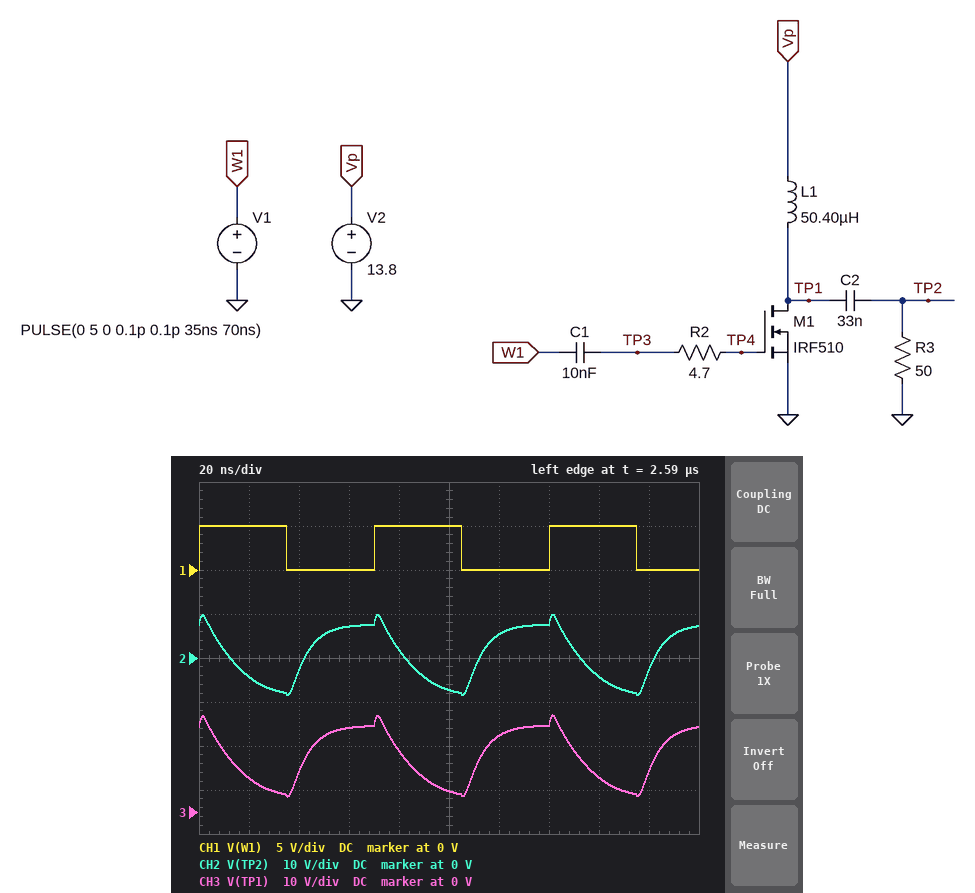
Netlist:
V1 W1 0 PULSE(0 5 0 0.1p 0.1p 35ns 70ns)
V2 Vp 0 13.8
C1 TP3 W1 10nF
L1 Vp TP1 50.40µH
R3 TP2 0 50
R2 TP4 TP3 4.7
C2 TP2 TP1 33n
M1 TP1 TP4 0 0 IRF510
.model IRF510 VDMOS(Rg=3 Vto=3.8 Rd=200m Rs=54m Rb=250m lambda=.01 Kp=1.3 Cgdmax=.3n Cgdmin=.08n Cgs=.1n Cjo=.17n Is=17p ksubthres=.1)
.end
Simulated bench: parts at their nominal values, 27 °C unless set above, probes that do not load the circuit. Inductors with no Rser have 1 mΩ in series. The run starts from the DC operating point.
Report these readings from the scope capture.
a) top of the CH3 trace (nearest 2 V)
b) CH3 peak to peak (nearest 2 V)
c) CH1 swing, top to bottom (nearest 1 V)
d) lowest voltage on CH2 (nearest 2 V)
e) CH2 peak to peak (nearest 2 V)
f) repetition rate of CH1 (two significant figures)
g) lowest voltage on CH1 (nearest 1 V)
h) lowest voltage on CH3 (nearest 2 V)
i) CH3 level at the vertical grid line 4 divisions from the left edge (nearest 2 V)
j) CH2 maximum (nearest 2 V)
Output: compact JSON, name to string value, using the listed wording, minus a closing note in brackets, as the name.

{"top of the CH3 trace": "22 V", "CH3 peak to peak": "18 V", "CH1 swing, top to bottom": "5 V", "lowest voltage on CH2": "-8 V", "CH2 peak to peak": "18 V", "repetition rate of CH1": "14 MHz", "lowest voltage on CH1": "0 V", "lowest voltage on CH3": "4 V", "CH3 level at the vertical grid line 4 divisions from the left edge": "14 V", "CH2 maximum": "10 V"}
